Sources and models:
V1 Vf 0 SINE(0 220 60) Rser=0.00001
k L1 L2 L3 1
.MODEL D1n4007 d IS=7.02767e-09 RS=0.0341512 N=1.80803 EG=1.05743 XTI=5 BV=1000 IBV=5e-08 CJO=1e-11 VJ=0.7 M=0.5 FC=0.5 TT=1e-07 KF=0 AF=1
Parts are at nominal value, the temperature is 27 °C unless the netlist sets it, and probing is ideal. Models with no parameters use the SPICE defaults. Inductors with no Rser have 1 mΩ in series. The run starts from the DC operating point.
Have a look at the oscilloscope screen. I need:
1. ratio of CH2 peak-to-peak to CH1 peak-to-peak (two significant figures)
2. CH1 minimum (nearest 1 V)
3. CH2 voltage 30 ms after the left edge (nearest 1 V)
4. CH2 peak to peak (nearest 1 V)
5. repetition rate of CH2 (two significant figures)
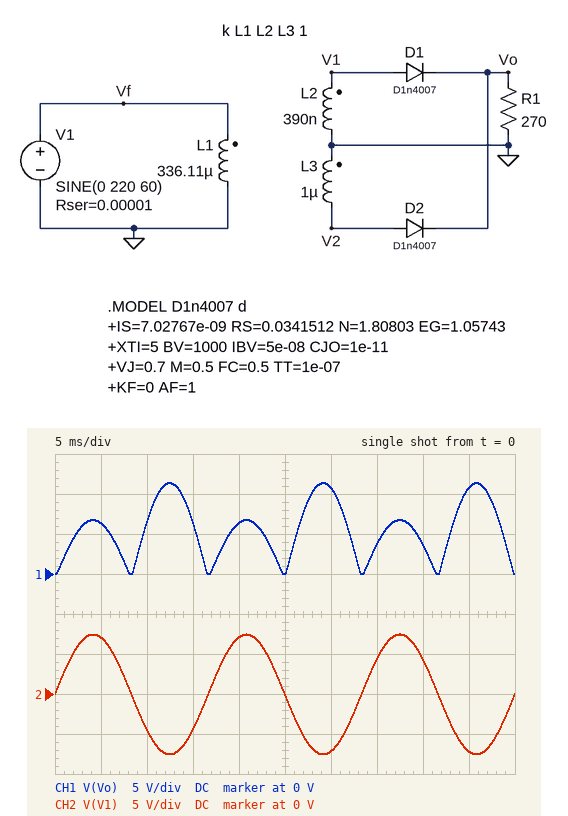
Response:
1.3
0 V
-7 V
15 V
60 Hz
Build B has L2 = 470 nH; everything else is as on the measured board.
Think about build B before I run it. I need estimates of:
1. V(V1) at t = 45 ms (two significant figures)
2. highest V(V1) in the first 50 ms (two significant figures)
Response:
-7.9 V
8.2 V
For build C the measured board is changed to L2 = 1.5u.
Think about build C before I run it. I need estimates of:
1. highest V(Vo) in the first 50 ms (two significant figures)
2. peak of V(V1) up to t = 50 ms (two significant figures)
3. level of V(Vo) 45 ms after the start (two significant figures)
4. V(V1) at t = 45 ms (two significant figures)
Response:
14 V
15 V
11 V
-14 V
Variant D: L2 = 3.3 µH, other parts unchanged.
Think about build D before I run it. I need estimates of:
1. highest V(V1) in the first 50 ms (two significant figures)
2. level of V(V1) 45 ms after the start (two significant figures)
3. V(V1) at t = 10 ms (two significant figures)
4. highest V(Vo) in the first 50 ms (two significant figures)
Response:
22 V
-21 V
-13 V
21 V
